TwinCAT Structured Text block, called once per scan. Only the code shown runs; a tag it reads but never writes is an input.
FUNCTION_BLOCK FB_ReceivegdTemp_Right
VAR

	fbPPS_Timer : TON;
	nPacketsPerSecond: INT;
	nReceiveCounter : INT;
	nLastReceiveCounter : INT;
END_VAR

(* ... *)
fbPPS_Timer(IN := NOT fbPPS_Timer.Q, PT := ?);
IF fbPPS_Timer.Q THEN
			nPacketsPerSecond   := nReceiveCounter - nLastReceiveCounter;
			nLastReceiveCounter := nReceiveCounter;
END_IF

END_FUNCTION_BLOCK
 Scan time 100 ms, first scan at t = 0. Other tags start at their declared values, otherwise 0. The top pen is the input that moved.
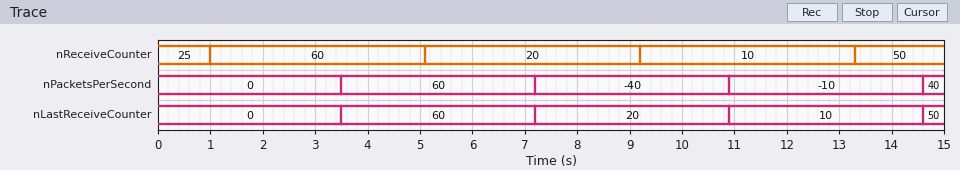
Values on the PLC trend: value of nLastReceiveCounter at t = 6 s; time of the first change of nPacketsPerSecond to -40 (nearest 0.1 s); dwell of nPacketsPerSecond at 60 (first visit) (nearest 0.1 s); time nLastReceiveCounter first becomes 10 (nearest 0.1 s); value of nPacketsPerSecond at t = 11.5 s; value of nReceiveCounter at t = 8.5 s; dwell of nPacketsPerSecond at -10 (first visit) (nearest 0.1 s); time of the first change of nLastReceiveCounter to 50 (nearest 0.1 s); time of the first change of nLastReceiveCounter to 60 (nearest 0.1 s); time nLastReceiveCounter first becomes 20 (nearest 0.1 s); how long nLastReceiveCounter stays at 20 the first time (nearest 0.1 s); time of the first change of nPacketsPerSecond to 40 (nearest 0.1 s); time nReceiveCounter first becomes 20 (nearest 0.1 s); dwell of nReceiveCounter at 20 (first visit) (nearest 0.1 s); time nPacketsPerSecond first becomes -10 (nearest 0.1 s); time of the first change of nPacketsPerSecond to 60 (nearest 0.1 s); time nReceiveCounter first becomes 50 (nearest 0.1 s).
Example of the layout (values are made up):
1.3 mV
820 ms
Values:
60
7.2 s
3.7 s
10.9 s
-10
20
3.7 s
14.6 s
3.5 s
7.2 s
3.7 s
14.6 s
5.1 s
4.1 s
10.9 s
3.5 s
13.3 s
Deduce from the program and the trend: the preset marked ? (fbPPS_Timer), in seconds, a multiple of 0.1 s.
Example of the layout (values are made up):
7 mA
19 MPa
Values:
3.5 s
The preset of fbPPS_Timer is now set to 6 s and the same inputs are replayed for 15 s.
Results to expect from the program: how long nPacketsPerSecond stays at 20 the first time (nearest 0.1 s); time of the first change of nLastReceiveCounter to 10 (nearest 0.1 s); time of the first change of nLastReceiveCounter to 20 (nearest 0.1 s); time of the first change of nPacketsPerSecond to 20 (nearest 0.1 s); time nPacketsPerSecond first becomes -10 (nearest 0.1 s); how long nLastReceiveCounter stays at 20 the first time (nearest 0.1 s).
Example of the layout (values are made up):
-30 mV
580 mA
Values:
6.2 s
12.2 s
6.0 s
6.0 s
12.2 s
6.2 s
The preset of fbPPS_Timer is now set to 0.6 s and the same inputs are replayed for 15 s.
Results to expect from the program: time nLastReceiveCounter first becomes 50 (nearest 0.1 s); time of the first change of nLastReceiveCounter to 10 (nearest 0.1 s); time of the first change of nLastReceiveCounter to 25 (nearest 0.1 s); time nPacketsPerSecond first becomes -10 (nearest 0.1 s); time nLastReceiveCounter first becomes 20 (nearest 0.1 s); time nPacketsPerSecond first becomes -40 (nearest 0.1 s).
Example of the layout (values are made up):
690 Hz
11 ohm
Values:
13.4 s
9.4 s
0.6 s
9.4 s
5.4 s
5.4 s
